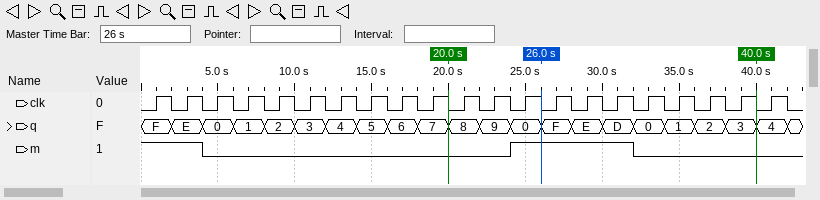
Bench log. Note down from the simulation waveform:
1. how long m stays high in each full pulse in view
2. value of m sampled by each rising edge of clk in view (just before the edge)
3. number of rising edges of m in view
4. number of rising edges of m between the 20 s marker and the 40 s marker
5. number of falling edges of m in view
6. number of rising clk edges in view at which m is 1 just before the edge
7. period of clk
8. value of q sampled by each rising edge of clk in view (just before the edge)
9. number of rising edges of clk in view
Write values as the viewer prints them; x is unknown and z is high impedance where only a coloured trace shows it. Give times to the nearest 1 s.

8 s
1 1 0 0 0 0 0 0 0 0 0 0 1 1 1 1 0 0 0 0 0
1
1
2
6
2 s
F, E, 0, 1, 2, 3, 4, 5, 6, 7, 8, 9, 0, F, E, D, 0, 1, 2, 3, 4
21
